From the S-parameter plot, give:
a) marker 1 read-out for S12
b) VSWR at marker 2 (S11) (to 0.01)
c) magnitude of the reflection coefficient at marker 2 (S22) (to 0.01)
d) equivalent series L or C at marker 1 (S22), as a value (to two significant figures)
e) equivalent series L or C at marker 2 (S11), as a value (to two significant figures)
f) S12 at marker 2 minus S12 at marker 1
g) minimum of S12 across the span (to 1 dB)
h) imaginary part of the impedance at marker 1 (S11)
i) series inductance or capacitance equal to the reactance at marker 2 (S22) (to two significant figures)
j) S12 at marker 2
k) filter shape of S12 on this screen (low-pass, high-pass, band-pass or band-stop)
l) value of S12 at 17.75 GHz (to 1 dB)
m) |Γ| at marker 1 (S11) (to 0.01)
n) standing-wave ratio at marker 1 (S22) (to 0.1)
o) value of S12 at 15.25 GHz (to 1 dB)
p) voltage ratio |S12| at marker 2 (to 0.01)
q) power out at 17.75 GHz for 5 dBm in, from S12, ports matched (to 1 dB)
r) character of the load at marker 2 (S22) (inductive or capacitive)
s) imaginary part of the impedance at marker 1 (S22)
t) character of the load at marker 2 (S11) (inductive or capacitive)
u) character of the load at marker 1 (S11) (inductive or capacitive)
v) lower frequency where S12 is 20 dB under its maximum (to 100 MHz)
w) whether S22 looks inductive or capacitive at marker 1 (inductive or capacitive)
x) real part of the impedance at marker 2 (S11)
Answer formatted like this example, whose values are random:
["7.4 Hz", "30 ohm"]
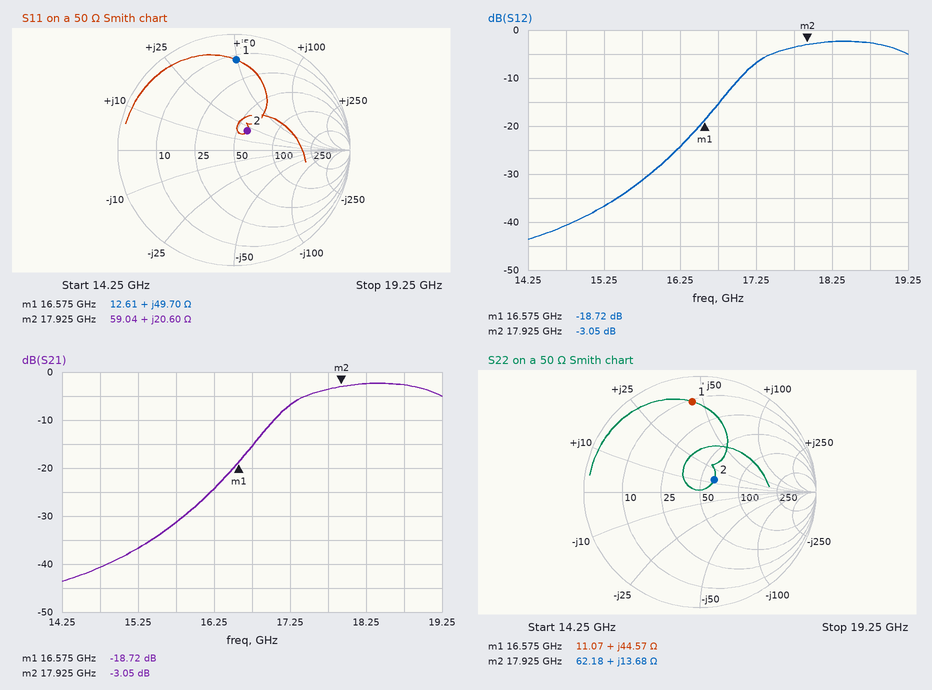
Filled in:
["-18.72 dB", "1.51", "0.16", "430 pH", "180 pH", "15.67 dB", "-44 dB", "+49.70 Ω", "120 pH", "-3.05 dB", "high-pass", "-4 dB", "0.78", "8.2", "-37 dB", "0.70", "1 dBm", "inductive", "+44.57 Ω", "inductive", "inductive", "16.4 GHz", "inductive", "59.04 Ω"]
